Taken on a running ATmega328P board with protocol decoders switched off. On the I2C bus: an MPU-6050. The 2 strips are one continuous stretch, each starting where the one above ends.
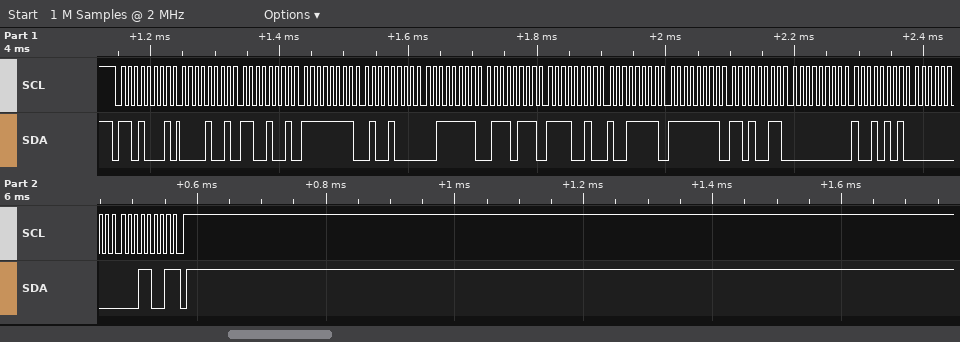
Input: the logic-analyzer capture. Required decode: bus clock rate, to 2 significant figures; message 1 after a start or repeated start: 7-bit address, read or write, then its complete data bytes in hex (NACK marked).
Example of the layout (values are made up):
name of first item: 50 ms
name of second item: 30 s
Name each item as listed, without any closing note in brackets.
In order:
bus clock rate, to 2 significant figures: 100 kHz
message 1 after a start or repeated start: 7-bit address, read or write, then its complete data bytes in hex: 0x68 read: 09 C9 FF 48 3F 77 F2 9F FF D3 00 95 00 19 NACK
